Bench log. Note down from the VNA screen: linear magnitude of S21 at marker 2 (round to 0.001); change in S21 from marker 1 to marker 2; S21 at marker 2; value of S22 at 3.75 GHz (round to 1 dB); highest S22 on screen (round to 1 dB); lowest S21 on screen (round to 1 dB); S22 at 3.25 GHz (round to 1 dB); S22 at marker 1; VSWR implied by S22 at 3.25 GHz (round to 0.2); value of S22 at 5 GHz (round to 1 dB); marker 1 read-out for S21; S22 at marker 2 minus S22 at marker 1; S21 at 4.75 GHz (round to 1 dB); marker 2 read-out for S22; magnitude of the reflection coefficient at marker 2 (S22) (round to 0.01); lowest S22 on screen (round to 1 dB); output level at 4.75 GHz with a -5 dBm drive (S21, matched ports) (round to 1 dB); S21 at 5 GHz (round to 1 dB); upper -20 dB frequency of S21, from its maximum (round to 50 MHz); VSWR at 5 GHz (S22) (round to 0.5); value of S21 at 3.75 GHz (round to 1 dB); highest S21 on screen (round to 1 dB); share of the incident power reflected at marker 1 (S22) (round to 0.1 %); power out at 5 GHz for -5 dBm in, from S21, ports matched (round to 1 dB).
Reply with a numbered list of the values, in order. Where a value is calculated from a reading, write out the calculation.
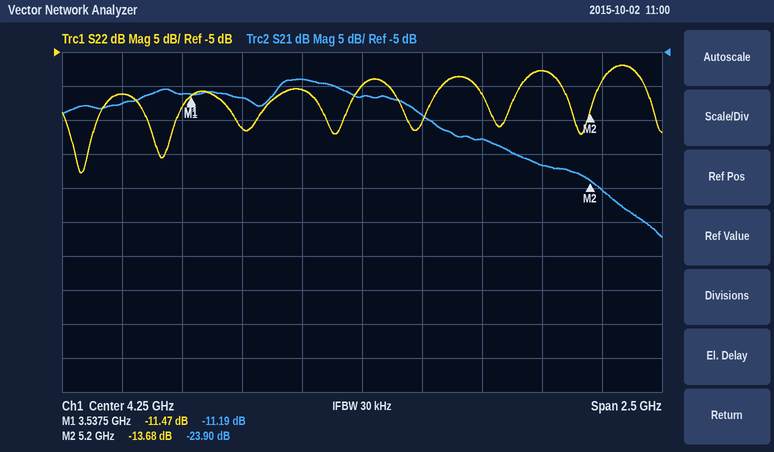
1. 10^(-23.9/20) ≈ 0.064
2. -23.9 − (-11.19) = -12.71 dB
3. -23.90 dB
4. -16 dB
5. -7 dB
6. -32 dB
7. -11 dB
8. -11.47 dB
9. |Γ| = 10^(-11/20) = 0.2818; VSWR = (1 + 0.2818)/(1 − 0.2818) ≈ 1.8
10. -8 dB
11. -11.19 dB
12. -13.68 − (-11.47) = -2.21 dB
13. -18 dB
14. -13.68 dB
15. 10^(-13.68/20) ≈ 0.21
16. -23 dB
17. -5 dBm + (-18 dB) = -23 dBm
18. -22 dB
19. 5.40 GHz
20. |Γ| = 10^(-8/20) = 0.3981; VSWR = (1 + 0.3981)/(1 − 0.3981) ≈ 2.32, so 2.5 to the nearest 0.5
21. -12 dB
22. -9 dB
23. 10^(-11.47/10) ≈ 7.1 %
24. -5 dBm + (-22 dB) = -27 dBm
